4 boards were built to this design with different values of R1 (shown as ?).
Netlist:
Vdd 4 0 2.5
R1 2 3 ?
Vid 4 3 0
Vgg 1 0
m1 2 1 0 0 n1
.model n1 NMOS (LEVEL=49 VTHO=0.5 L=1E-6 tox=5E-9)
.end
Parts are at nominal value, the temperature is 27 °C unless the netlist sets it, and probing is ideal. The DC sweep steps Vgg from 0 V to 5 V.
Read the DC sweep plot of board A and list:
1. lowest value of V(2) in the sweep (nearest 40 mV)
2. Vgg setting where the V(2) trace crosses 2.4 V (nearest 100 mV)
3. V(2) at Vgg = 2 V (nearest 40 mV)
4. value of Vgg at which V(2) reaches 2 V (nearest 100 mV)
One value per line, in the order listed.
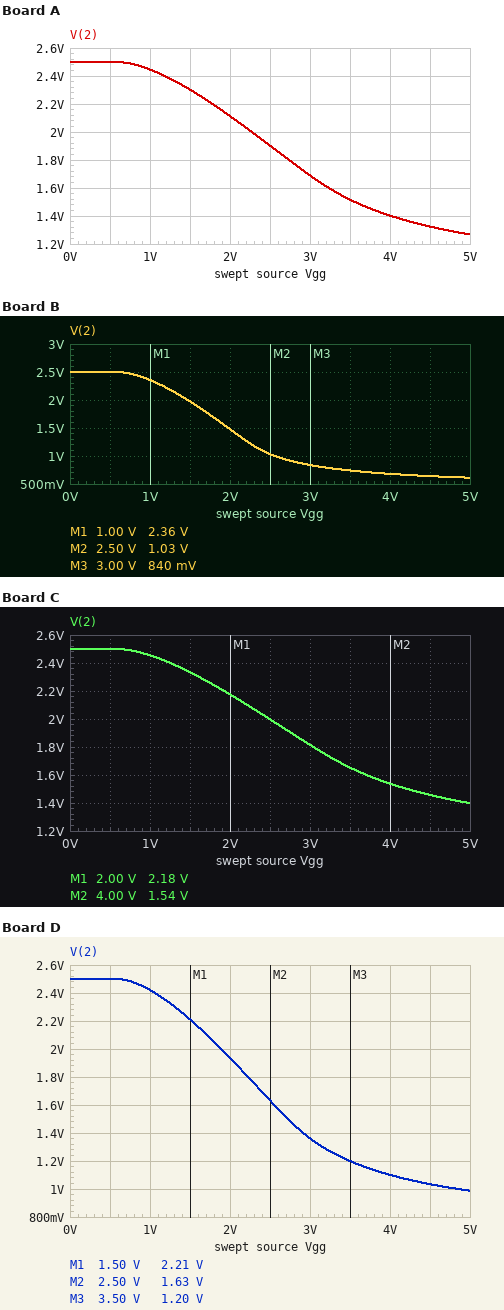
1.28 V
1.2 V
2.12 V
2.3 V
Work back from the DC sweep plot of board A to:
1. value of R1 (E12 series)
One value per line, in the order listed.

560 Ω
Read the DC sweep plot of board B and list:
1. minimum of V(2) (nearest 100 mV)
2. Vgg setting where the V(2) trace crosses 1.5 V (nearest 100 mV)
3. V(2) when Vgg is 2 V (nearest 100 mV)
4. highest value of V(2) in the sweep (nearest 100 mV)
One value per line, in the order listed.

600 mV
2.0 V
1.5 V
2.5 V
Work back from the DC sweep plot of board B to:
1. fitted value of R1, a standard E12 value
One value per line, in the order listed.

1.5 kΩ
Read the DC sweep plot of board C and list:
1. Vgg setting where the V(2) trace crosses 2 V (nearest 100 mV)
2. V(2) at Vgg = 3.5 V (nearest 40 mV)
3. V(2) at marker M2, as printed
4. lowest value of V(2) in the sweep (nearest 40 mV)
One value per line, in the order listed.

2.5 V
1.64 V
1.54 V
1.40 V
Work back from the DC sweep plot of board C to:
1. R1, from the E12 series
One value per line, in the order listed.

470 Ω
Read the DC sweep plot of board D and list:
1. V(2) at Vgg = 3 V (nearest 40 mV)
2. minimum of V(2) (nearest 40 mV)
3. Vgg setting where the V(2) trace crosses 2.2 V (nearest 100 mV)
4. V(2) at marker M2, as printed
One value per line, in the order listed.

1.36 V
1.00 V
1.5 V
1.63 V
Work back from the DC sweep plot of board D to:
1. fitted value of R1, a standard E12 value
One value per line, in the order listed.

820 Ω
